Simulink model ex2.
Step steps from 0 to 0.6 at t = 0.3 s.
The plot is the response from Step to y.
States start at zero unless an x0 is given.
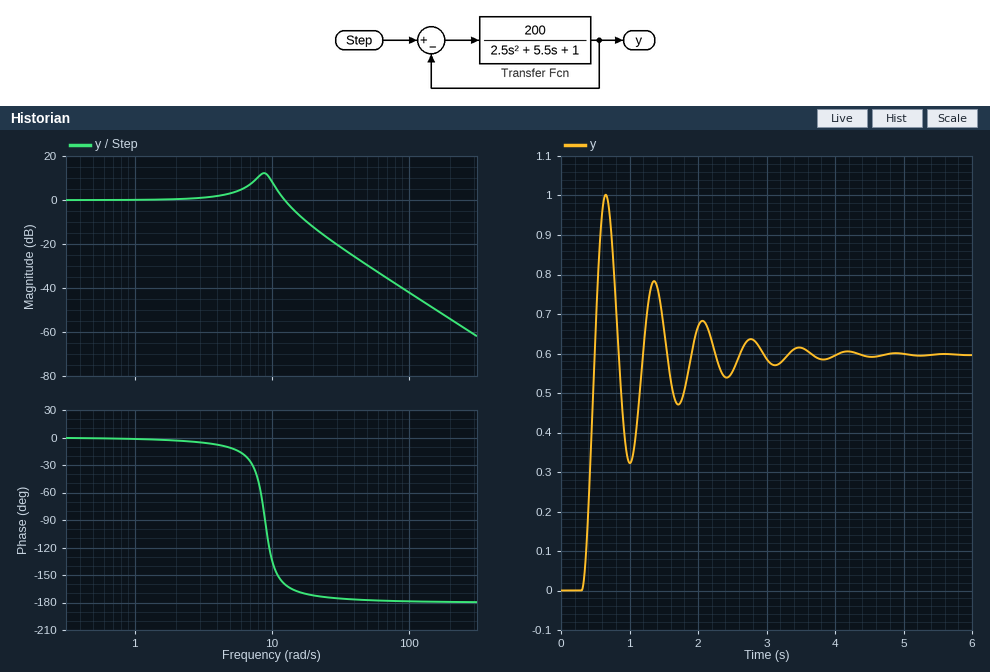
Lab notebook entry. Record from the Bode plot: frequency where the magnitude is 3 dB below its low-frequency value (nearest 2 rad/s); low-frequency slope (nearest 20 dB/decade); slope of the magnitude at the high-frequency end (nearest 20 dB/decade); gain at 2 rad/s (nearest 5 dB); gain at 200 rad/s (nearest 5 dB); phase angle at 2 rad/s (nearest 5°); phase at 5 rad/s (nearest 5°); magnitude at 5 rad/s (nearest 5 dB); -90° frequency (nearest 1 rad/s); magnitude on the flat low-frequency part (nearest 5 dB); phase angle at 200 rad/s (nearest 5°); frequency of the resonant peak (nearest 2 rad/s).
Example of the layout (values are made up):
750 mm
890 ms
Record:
14 rad/s
0 dB/decade
-40 dB/decade
0 dB
-55 dB
-5°
-10°
5 dB
9 rad/s
0 dB
-180°
8 rad/s
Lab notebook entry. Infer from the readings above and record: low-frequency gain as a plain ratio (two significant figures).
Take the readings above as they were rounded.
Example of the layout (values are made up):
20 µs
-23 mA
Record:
1.0
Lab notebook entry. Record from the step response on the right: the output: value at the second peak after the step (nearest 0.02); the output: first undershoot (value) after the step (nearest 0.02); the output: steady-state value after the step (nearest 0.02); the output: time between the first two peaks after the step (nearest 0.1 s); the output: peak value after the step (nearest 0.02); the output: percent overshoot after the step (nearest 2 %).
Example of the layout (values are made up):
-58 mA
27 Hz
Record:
0.78
0.32
0.60
0.7 s
1.00
68 %
